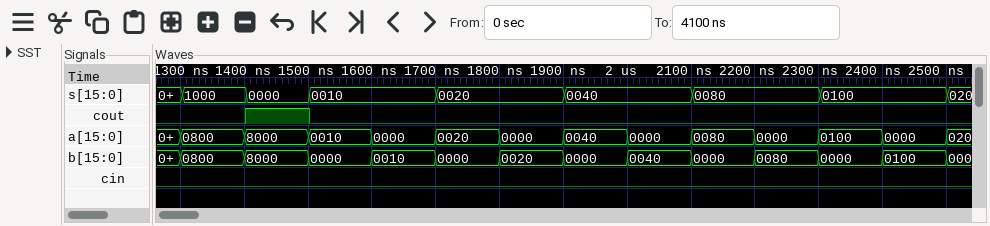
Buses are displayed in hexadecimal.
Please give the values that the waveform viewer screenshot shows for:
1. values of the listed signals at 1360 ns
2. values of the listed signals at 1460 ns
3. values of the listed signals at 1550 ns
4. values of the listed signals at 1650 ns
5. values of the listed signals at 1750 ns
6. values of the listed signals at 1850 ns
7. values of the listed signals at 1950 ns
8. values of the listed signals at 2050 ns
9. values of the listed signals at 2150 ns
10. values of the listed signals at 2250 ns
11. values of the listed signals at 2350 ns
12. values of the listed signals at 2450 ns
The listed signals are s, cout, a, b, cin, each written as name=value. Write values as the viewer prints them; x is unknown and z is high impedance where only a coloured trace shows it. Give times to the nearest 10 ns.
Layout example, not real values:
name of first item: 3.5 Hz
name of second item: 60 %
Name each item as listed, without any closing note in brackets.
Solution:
values of the listed signals at 1360 ns: s=1000, cout=0, a=0800, b=0800, cin=0
values of the listed signals at 1460 ns: s=0000, cout=1, a=8000, b=8000, cin=0
values of the listed signals at 1550 ns: s=0010, cout=0, a=0010, b=0000, cin=0
values of the listed signals at 1650 ns: s=0010, cout=0, a=0000, b=0010, cin=0
values of the listed signals at 1750 ns: s=0020, cout=0, a=0020, b=0000, cin=0
values of the listed signals at 1850 ns: s=0020, cout=0, a=0000, b=0020, cin=0
values of the listed signals at 1950 ns: s=0040, cout=0, a=0040, b=0000, cin=0
values of the listed signals at 2050 ns: s=0040, cout=0, a=0000, b=0040, cin=0
values of the listed signals at 2150 ns: s=0080, cout=0, a=0080, b=0000, cin=0
values of the listed signals at 2250 ns: s=0080, cout=0, a=0000, b=0080, cin=0
values of the listed signals at 2350 ns: s=0100, cout=0, a=0100, b=0000, cin=0
values of the listed signals at 2450 ns: s=0100, cout=0, a=0000, b=0100, cin=0
